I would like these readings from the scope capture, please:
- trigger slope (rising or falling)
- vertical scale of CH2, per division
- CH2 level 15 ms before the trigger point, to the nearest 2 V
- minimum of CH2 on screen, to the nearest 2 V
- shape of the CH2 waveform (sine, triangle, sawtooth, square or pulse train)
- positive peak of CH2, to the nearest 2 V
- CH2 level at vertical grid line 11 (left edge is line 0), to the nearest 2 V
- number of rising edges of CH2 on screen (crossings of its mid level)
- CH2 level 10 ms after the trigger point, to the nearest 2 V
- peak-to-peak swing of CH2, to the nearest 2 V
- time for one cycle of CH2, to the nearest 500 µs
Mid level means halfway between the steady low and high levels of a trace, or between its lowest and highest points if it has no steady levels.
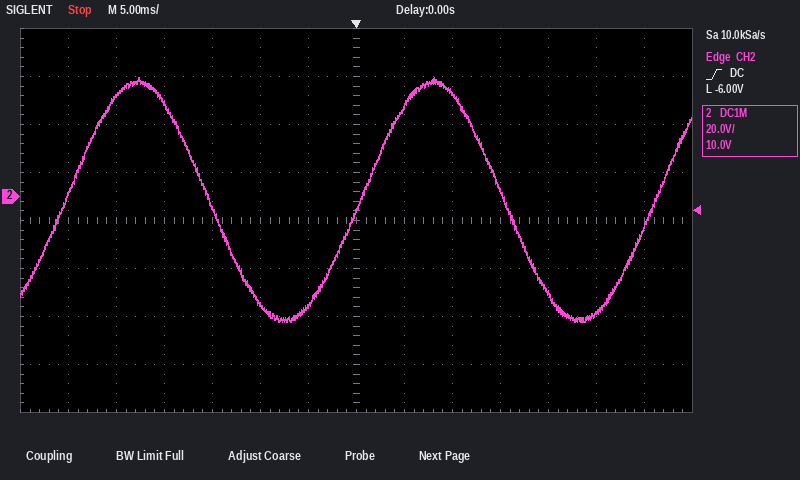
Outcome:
rising
20 V
-4 V
-52 V
sine
50 V
-40 V
3
44 V
102 V
30.5 ms
